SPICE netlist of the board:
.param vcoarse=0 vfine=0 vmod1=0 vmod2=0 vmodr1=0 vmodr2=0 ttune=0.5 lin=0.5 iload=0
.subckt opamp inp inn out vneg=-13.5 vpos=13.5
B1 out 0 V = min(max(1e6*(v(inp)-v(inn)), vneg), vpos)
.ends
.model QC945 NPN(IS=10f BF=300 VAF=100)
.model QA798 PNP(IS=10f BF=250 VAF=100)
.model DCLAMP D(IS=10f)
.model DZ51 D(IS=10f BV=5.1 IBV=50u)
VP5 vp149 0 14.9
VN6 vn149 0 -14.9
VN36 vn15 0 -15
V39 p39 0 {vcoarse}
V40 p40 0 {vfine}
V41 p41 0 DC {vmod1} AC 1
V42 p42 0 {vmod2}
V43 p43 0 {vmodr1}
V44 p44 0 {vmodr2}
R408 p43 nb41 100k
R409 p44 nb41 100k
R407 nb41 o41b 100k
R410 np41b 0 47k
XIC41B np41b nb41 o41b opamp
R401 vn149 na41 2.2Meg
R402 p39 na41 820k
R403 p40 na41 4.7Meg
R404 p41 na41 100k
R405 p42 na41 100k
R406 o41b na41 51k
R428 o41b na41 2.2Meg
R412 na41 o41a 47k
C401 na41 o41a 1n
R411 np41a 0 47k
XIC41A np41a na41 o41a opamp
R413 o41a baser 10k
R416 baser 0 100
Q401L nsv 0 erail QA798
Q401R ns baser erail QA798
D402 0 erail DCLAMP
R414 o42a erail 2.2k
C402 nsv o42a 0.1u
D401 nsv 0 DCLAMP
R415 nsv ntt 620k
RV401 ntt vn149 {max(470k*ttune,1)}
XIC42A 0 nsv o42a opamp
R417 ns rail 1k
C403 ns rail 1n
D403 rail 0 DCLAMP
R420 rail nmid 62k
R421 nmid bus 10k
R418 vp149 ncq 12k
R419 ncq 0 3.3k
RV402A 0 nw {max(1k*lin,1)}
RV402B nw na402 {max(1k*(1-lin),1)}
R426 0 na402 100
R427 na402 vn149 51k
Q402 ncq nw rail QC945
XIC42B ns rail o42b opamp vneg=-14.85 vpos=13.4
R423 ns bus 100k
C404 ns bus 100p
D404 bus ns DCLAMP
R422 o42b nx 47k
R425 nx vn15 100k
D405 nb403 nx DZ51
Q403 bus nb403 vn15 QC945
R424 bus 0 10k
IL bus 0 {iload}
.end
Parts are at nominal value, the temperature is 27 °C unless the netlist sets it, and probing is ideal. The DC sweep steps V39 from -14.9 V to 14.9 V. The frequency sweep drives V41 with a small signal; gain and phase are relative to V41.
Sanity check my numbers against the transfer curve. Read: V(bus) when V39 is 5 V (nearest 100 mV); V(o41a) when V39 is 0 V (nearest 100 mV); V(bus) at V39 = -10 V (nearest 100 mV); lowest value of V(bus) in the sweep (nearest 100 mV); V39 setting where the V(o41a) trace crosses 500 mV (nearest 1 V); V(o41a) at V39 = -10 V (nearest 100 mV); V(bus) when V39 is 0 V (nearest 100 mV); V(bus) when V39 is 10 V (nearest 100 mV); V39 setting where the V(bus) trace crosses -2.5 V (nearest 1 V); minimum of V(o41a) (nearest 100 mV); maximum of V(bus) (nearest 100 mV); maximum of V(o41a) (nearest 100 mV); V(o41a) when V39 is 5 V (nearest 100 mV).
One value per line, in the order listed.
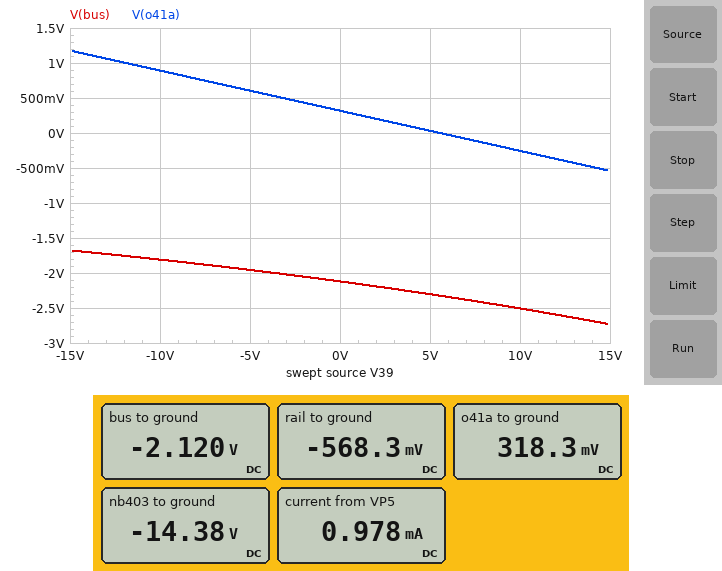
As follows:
-2.3 V
300 mV
-1.8 V
-2.7 V
-3 V
900 mV
-2.1 V
-2.5 V
10 V
-500 mV
-1.7 V
1.2 V
0 V
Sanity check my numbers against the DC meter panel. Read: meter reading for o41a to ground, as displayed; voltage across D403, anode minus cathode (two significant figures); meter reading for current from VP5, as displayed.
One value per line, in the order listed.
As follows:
318.3 mV
-570 mV
0.978 mA
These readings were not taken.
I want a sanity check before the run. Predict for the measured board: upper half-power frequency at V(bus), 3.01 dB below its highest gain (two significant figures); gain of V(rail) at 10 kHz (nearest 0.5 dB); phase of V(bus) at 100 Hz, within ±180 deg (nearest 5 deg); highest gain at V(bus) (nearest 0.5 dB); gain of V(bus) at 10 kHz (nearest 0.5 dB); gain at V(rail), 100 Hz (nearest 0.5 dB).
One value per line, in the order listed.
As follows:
640 Hz
-61.5 dB
170 deg
-11.0 dB
-26.0 dB
-47.0 dB
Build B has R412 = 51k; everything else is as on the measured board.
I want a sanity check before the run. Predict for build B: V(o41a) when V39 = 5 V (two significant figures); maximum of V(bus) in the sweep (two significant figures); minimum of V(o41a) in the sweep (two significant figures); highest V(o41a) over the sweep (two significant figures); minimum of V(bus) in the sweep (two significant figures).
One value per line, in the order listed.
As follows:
34 mV
-1.6 V
-580 mV
1.3 V
-2.8 V
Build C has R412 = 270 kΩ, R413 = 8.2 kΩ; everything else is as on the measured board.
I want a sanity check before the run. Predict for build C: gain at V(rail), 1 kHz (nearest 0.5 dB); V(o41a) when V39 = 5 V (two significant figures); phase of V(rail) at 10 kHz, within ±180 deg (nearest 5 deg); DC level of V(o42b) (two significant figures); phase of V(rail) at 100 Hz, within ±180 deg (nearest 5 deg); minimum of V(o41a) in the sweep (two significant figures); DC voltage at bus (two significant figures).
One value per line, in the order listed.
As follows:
-37.5 dB
180 mV
60 deg
-6.8 V
165 deg
-3.1 V
-1.3 V
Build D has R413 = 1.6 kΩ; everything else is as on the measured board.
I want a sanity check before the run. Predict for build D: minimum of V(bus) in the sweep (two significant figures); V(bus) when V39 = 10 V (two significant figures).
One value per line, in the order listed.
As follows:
-6.5 V
-3.7 V
